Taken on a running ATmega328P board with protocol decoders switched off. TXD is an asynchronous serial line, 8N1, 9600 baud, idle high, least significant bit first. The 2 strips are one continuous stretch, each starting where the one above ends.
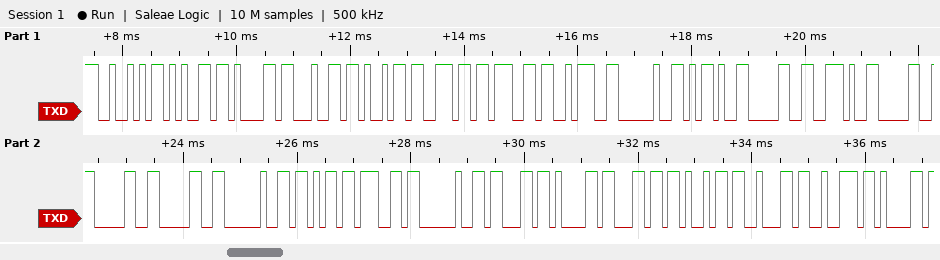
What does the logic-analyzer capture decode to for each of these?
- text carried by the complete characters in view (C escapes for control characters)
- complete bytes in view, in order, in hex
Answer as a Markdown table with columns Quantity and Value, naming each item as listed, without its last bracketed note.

| Quantity | Value |
|---|---|
| text carried by the complete characters in view | "Reading: -0.000 kg calibra" |
| complete bytes in view, in order, in hex | 52 65 61 64 69 6E 67 3A 20 2D 30 2E 30 30 30 20 6B 67 20 63 61 6C 69 62 72 61 |
